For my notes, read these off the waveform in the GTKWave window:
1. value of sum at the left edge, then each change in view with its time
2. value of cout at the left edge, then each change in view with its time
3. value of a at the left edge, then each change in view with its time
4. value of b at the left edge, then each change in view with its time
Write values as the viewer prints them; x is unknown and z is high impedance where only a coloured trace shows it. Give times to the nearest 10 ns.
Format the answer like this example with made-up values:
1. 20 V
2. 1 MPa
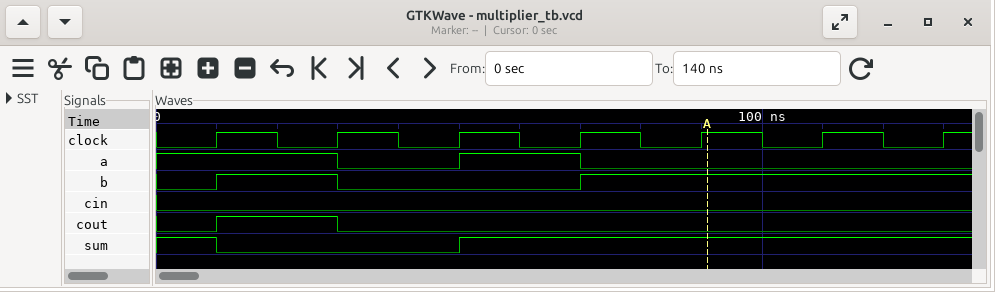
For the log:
1. 1, 0 at 10 ns, 1 at 50 ns
2. 0, 1 at 10 ns, 0 at 30 ns
3. 1, 0 at 30 ns, 1 at 50 ns, 0 at 70 ns
4. 0, 1 at 10 ns, 0 at 30 ns, 1 at 70 ns
